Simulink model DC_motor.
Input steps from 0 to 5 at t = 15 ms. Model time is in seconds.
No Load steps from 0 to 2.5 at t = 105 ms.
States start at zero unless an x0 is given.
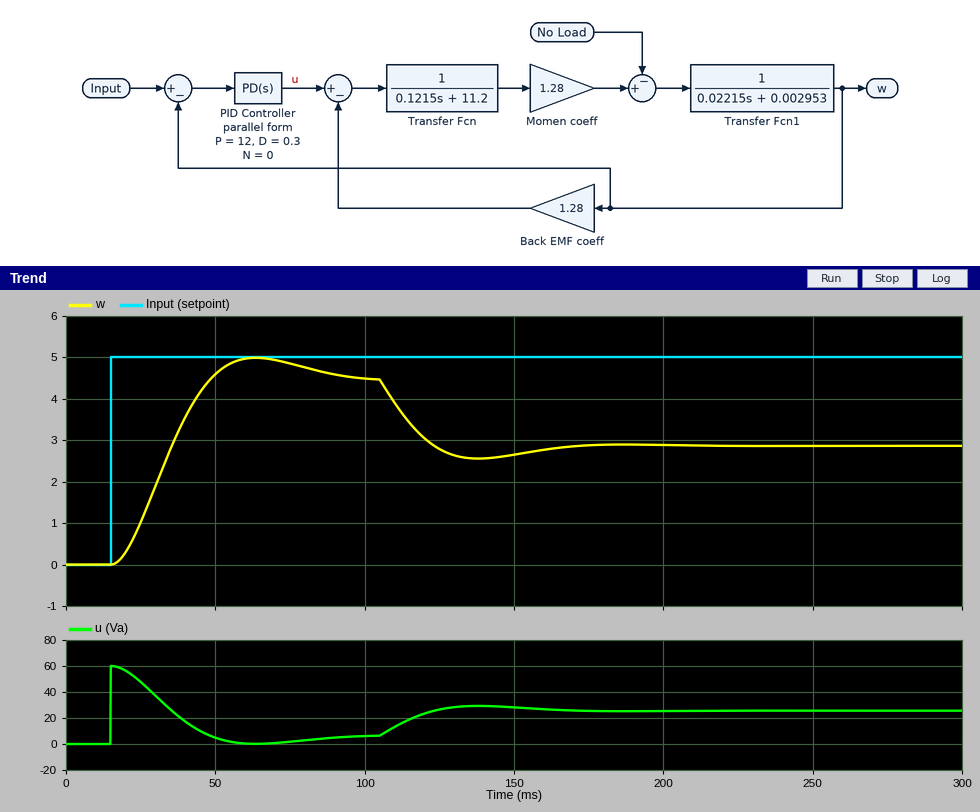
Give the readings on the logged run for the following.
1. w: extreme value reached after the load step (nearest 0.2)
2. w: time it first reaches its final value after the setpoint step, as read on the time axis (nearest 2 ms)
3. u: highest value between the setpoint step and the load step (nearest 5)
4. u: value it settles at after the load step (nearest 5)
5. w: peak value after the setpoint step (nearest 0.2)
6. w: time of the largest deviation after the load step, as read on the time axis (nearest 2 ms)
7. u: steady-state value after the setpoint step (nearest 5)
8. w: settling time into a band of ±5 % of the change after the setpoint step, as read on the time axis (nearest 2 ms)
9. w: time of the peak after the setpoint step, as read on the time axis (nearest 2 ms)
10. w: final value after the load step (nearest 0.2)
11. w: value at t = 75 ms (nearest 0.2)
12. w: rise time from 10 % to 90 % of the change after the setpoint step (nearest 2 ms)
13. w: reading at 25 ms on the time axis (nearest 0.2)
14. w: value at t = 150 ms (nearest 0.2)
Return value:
2.6
48 ms
60
25
5.0
138 ms
5
82 ms
64 ms
2.8
4.8
22 ms
1.0
2.6
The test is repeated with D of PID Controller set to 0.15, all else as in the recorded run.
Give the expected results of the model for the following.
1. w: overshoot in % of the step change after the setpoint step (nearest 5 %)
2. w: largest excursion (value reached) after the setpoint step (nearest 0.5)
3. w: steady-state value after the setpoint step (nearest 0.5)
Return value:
10 %
5.0
4.5
